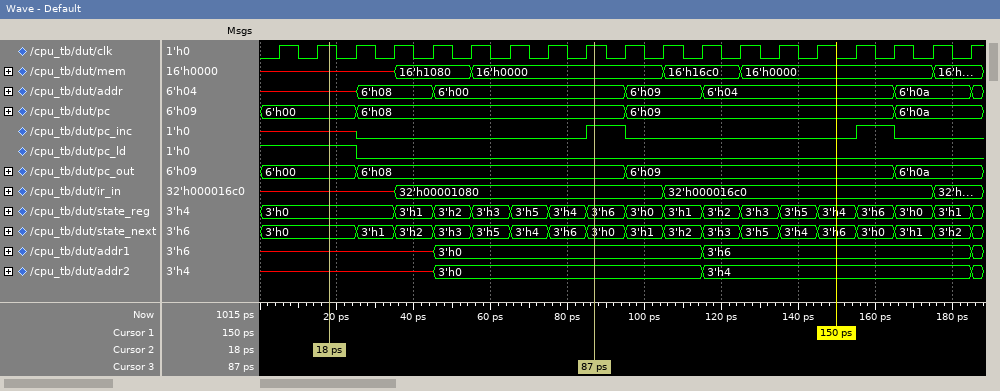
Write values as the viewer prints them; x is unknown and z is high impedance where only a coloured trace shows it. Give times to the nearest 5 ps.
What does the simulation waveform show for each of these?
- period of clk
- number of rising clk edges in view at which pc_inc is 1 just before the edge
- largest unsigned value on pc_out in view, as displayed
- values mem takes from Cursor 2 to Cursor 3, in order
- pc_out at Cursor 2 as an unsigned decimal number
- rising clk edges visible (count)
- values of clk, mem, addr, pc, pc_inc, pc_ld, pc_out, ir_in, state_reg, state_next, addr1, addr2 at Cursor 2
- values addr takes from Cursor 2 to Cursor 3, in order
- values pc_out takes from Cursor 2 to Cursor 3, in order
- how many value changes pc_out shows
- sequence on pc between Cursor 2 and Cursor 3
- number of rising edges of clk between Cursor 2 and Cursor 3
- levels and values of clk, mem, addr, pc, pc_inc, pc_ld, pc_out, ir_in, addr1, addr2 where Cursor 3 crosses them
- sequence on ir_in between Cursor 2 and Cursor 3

10 ps
2
6'h0a
x, 16'h1080, 16'h0000
0
19
clk=1, mem=x, addr=x, pc=6'h00, pc_inc=x, pc_ld=1, pc_out=6'h00, ir_in=x, state_reg=3'h0, state_next=3'h0, addr1=x, addr2=x
x, 6'h08, 6'h00
6'h00, 6'h08
3
6'h00, 6'h08
7
clk=1, mem=16'h0000, addr=6'h00, pc=6'h08, pc_inc=1, pc_ld=0, pc_out=6'h08, ir_in=32'h00001080, addr1=3'h0, addr2=3'h0
x, 32'h00001080
